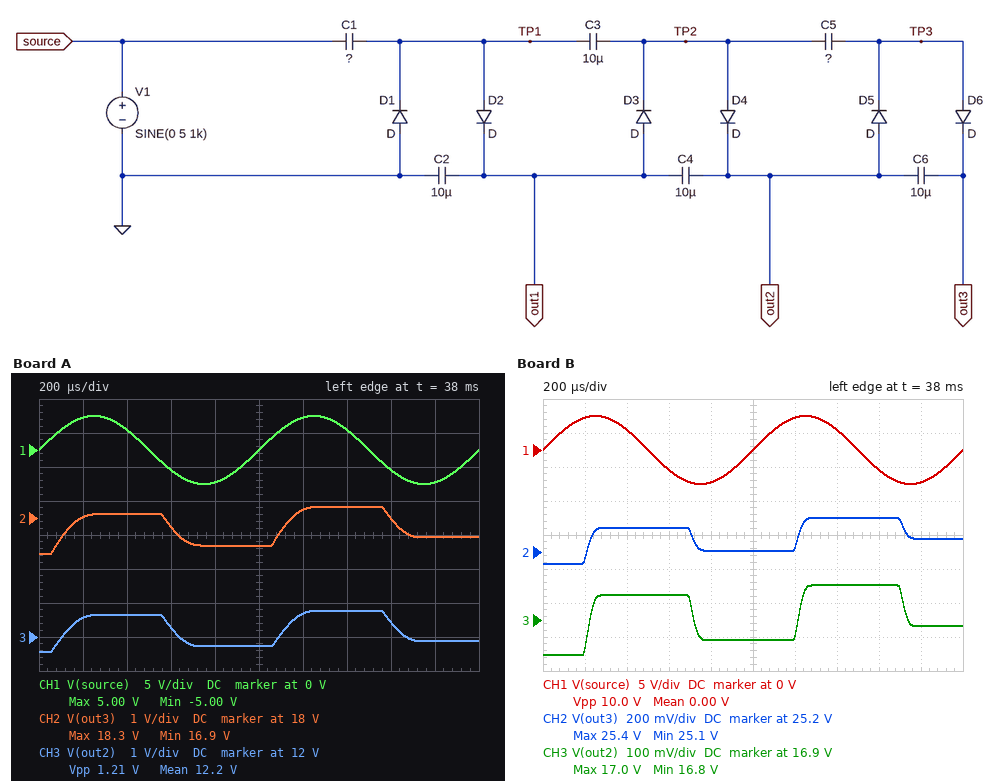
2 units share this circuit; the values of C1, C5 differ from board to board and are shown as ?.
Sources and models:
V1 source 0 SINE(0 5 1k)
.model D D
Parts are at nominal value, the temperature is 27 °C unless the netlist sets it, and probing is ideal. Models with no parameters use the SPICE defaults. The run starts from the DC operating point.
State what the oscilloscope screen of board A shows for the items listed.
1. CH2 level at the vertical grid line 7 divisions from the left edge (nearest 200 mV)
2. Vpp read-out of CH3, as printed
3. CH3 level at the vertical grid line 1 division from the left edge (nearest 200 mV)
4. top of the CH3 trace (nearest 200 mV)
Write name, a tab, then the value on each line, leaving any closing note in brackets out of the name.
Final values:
CH2 level at the vertical grid line 7 divisions from the left edge	18.4 V
Vpp read-out of CH3, as printed	1.21 V
CH3 level at the vertical grid line 1 division from the left edge	12.6 V
top of the CH3 trace	12.8 V
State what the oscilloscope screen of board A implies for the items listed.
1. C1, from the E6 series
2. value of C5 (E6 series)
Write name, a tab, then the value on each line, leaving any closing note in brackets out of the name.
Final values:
C1, from the E6 series	3.3 µF
value of C5	33 µF
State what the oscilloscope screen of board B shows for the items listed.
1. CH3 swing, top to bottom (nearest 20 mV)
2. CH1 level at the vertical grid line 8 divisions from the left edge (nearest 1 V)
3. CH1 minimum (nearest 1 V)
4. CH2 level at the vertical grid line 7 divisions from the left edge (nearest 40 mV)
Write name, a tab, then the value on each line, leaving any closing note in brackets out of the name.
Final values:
CH3 swing, top to bottom	200 mV
CH1 level at the vertical grid line 8 divisions from the left edge	-3 V
CH1 minimum	-5 V
CH2 level at the vertical grid line 7 divisions from the left edge	25.40 V
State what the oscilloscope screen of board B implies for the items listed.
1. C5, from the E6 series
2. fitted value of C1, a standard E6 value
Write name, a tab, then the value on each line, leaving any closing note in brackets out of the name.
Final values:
C5, from the E6 series	4.7 µF
fitted value of C1, a standard E6 value	15 µF
